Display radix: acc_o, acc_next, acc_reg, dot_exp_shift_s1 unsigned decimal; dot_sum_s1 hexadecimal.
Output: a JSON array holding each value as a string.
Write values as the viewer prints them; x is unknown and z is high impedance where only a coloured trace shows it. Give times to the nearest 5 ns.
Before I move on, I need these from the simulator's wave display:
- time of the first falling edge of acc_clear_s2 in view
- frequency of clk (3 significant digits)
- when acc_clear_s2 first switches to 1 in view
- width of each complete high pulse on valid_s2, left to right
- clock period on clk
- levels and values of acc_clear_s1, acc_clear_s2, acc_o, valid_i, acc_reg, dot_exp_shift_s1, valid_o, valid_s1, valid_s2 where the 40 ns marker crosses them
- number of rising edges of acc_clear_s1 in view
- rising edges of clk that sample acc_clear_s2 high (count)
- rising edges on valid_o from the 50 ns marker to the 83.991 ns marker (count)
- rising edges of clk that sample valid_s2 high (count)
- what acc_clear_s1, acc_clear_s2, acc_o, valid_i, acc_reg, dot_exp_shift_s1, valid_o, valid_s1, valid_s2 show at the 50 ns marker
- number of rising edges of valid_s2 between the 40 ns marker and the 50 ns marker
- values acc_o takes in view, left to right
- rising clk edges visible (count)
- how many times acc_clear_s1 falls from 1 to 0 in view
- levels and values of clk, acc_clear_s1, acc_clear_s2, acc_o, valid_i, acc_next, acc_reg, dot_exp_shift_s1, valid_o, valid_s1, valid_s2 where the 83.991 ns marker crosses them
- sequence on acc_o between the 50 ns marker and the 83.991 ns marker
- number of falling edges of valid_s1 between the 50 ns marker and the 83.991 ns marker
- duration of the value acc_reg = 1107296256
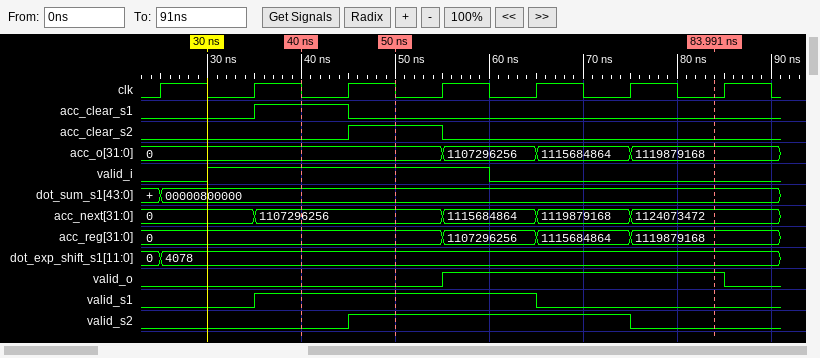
["55 ns", "100 MHz", "45 ns", "30 ns", "10 ns", "acc_clear_s1=1, acc_clear_s2=0, acc_o=0, valid_i=1, acc_reg=0, dot_exp_shift_s1=4078, valid_o=0, valid_s1=1, valid_s2=0", "1", "1", "1", "3", "acc_clear_s1=0, acc_clear_s2=1, acc_o=0, valid_i=1, acc_reg=0, dot_exp_shift_s1=4078, valid_o=0, valid_s1=1, valid_s2=1", "1", "0, 1107296256, 1115684864, 1119879168", "7", "1", "clk=0, acc_clear_s1=0, acc_clear_s2=0, acc_o=1119879168, valid_i=0, acc_next=1124073472, acc_reg=1119879168, dot_exp_shift_s1=4078, valid_o=1, valid_s1=0, valid_s2=0", "0, 1107296256, 1115684864, 1119879168", "1", "10 ns"]
